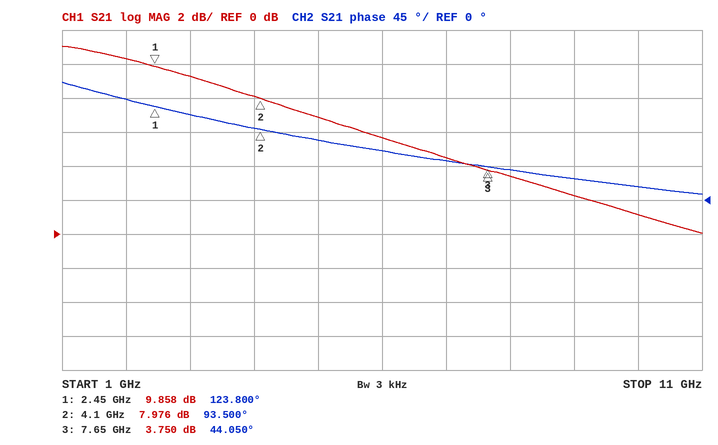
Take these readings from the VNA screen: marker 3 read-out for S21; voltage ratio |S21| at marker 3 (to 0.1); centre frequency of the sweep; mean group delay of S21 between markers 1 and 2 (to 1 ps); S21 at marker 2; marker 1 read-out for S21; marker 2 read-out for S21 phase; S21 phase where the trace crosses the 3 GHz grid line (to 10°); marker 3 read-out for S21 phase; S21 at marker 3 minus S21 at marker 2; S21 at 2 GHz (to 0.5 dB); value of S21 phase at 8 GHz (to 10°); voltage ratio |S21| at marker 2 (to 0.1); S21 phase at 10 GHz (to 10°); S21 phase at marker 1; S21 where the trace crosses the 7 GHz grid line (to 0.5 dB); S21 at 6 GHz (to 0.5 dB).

3.750 dB
1.5
6 GHz
51 ps
7.976 dB
9.858 dB
93.500°
110°
44.050°
-4.226 dB
10.5 dB
40°
2.5
20°
123.800°
4.5 dB
5.5 dB
